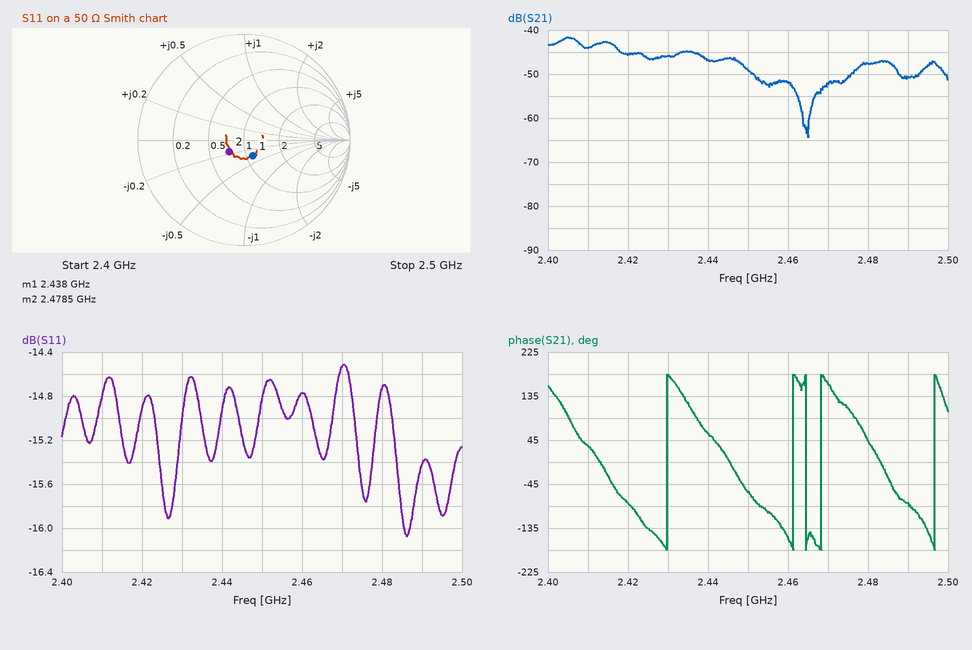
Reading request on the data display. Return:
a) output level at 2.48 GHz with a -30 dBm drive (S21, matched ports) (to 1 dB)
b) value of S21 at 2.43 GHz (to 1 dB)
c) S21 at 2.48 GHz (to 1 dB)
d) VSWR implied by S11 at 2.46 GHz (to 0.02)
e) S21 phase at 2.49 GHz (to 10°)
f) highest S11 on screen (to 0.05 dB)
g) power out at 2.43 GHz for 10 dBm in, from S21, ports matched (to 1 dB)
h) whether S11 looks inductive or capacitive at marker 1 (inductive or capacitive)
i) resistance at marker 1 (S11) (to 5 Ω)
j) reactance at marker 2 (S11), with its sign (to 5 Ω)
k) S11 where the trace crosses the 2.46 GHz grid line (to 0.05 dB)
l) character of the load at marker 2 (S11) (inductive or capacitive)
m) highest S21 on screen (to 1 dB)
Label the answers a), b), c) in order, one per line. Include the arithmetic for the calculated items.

a) -30 dBm + (-48 dB) = -78 dBm
b) -46 dB
c) -48 dB
d) |Γ| = 10^(-14.75/20) = 0.1830; VSWR = (1 + 0.1830)/(1 − 0.1830) ≈ 1.45, so 1.44 to the nearest 0.02
e) -80°
f) -14.50 dB
g) 10 dBm + (-46 dB) = -36 dBm
h) capacitive
i) 55 Ω
j) -10 Ω
k) -14.75 dB
l) capacitive
m) -42 dB
